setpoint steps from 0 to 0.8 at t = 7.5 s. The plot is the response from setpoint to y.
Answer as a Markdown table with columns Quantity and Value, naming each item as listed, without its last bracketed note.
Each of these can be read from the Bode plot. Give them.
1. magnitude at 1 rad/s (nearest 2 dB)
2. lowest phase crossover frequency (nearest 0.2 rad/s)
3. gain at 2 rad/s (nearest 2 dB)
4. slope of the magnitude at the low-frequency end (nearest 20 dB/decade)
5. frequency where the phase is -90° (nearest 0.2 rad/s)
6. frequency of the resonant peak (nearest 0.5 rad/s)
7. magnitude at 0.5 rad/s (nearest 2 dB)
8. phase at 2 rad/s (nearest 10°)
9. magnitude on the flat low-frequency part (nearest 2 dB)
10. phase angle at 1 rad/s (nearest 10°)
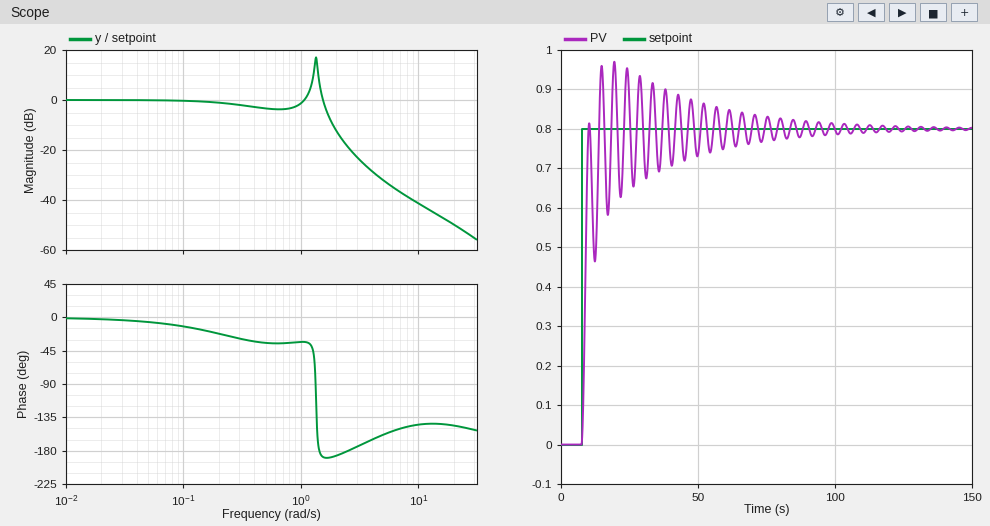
| Quantity | Value |
|---|---|
| magnitude at 1 rad/s | -2 dB |
| lowest phase crossover frequency | 1.4 rad/s |
| gain at 2 rad/s | -12 dB |
| slope of the magnitude at the low-frequency end | 0 dB/decade |
| frequency where the phase is -90° | 1.4 rad/s |
| frequency of the resonant peak | 1.5 rad/s |
| magnitude at 0.5 rad/s | -4 dB |
| phase at 2 rad/s | -190° |
| magnitude on the flat low-frequency part | 0 dB |
| phase angle at 1 rad/s | -30° |
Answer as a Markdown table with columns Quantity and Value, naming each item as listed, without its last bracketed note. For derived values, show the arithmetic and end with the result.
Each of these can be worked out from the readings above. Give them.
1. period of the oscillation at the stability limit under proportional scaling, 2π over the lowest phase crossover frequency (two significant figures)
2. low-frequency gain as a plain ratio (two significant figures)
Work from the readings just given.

| Quantity | Value |
|---|---|
| period of the oscillation at the stability limit under proportional scaling, 2π over the lowest phase crossover frequency | 2π / 1.4 = 4.5 s |
| low-frequency gain as a plain ratio | 10^(0 / 20) = 1.0 |
